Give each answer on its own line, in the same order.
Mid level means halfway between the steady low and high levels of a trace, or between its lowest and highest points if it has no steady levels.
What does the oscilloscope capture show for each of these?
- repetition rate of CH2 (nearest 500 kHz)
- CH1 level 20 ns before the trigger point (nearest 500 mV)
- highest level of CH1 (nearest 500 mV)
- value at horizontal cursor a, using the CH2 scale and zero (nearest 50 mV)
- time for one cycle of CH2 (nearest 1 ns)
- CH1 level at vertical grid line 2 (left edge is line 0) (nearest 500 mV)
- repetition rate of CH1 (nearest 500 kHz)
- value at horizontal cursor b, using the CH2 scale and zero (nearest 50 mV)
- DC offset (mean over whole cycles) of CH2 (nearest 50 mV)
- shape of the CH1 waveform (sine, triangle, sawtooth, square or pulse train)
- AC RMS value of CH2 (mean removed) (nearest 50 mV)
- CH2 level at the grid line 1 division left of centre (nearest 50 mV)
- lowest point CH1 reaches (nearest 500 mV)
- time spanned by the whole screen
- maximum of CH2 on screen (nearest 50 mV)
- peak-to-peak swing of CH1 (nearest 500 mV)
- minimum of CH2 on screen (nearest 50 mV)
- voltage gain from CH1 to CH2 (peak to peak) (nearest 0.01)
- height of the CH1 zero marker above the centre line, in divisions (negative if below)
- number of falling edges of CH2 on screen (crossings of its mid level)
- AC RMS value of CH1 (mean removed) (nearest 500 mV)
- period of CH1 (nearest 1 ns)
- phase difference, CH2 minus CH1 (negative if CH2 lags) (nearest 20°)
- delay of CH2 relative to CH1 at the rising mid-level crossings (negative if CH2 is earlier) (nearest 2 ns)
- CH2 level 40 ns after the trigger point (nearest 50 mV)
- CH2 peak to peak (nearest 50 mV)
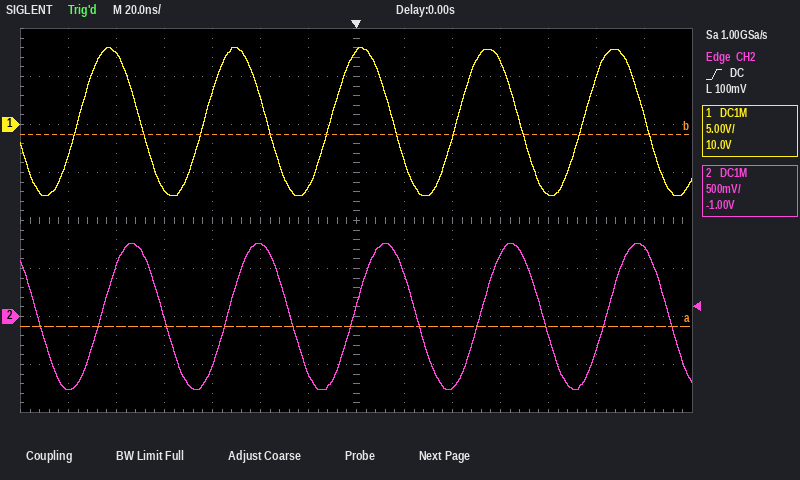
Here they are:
19.0 MHz
-6.5 V
8.0 V
-100 mV
53 ns
7.5 V
19.0 MHz
1.90 V
0 mV
sine
550 mV
-600 mV
-7.5 V
280 ns
750 mV
15.5 V
-750 mV
0.10
+2.0 div
6
5.5 V
53 ns
-60°
+10 ns
-750 mV
1.50 V
